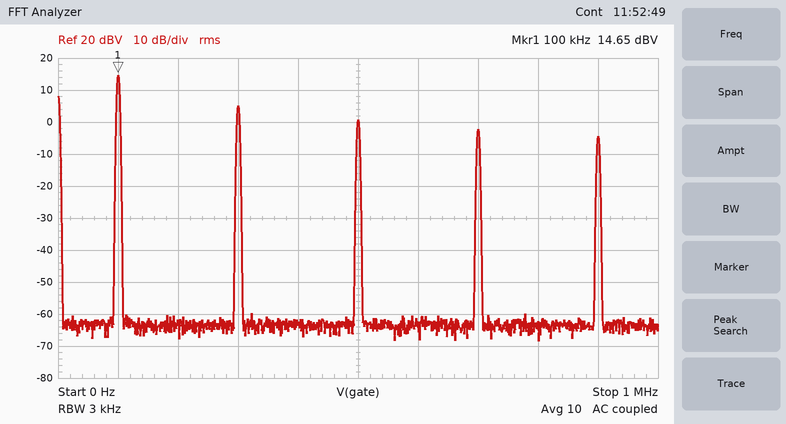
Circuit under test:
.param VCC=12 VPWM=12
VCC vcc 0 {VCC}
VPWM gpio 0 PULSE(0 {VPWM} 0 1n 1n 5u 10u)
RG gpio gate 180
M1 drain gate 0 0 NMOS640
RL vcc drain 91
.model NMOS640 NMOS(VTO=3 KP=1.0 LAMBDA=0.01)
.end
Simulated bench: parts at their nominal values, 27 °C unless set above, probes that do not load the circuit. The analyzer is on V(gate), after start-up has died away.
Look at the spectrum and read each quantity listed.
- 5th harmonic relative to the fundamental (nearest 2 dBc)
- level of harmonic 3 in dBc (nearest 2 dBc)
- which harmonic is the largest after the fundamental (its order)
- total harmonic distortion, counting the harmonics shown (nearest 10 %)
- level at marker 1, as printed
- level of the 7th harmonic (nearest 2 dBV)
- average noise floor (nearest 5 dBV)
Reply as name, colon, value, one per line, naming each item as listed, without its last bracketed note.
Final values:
5th harmonic relative to the fundamental: -14 dBc
level of harmonic 3 in dBc: -10 dBc
which harmonic is the largest after the fundamental: 3
total harmonic distortion, counting the harmonics shown: 40 %
level at marker 1, as printed: 14.65 dBV
level of the 7th harmonic: -2 dBV
average noise floor: -65 dBV
